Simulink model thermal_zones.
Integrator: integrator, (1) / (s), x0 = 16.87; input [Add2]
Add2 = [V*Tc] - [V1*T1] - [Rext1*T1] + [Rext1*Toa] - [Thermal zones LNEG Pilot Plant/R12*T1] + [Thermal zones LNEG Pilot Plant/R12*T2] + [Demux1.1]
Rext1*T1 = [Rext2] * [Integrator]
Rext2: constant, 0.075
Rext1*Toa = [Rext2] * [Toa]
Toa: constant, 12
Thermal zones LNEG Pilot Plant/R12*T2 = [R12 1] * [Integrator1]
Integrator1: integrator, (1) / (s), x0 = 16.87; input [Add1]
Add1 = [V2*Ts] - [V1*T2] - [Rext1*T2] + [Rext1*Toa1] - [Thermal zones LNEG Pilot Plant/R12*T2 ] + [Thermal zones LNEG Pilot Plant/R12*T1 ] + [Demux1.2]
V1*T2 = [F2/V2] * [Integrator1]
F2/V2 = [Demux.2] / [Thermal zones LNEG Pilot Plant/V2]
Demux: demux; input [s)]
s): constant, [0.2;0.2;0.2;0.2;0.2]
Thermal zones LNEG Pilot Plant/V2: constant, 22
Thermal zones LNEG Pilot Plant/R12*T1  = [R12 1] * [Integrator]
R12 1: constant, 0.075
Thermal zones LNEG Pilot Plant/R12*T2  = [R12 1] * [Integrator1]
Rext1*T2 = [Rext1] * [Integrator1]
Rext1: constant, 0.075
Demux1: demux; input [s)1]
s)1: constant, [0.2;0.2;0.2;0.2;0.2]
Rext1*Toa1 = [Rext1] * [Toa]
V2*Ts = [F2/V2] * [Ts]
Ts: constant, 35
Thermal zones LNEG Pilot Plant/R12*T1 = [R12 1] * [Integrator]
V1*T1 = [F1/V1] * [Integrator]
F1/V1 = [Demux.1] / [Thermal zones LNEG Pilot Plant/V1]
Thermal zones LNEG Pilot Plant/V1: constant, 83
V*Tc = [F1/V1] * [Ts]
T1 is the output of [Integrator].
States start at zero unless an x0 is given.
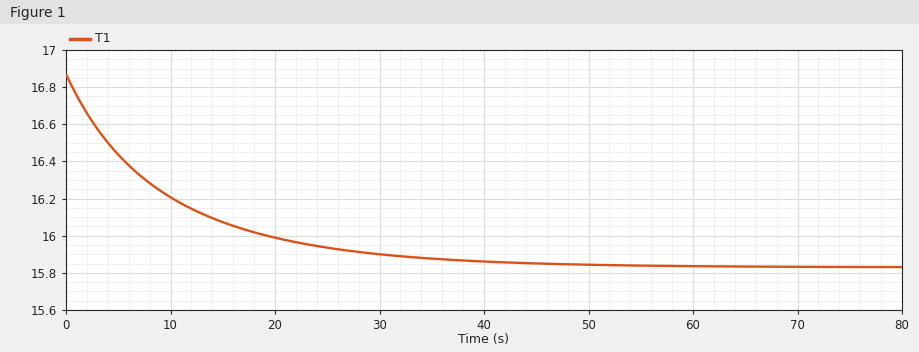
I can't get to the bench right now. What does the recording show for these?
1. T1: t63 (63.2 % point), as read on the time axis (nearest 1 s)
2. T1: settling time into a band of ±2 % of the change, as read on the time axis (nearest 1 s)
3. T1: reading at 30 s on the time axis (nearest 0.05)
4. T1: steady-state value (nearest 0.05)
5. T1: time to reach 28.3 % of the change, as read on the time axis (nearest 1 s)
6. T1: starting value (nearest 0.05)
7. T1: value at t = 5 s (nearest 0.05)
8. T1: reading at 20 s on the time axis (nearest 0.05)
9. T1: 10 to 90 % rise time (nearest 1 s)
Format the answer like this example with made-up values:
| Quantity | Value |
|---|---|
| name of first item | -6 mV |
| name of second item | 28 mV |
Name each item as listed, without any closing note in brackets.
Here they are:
| Quantity | Value |
|---|---|
| T1: t63 (63.2 % point), as read on the time axis | 10 s |
| T1: settling time into a band of ±2 % of the change, as read on the time axis | 45 s |
| T1: reading at 30 s on the time axis | 15.90 |
| T1: steady-state value | 15.85 |
| T1: time to reach 28.3 % of the change, as read on the time axis | 3 s |
| T1: starting value | 16.85 |
| T1: value at t = 5 s | 16.45 |
| T1: reading at 20 s on the time axis | 16.00 |
| T1: 10 to 90 % rise time | 24 s |
